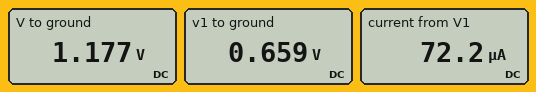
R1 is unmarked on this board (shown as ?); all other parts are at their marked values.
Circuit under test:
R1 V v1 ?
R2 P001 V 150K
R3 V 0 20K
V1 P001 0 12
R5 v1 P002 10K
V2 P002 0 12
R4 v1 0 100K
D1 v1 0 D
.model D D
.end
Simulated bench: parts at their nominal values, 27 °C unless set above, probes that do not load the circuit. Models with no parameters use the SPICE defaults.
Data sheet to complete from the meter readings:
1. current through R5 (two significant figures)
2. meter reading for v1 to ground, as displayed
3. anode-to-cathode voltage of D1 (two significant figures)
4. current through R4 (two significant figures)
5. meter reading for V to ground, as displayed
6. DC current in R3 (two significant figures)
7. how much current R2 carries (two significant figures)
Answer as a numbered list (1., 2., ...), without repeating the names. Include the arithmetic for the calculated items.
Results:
1. (12 V - 659 mV) / 10 kΩ = 1.1 mA
2. 0.659 V
3. 659 mV = 660 mV
4. (659 mV) / 100 kΩ = 6.6 µA
5. 1.177 V
6. (1.177 V) / 20 kΩ = 59 µA
7. (12 V - 1.177 V) / 150 kΩ = 72 µA
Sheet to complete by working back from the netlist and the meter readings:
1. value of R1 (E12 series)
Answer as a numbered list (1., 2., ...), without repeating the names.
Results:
1. 39 kΩ
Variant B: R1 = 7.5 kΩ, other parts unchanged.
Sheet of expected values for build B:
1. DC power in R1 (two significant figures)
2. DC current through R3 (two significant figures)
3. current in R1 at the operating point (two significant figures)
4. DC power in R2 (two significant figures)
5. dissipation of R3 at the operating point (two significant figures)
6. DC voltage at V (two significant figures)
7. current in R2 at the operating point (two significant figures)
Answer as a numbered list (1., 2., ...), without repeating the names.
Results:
1. 6.7 µW
2. 44 µA
3. 30 µA
4. 820 µW
5. 39 µW
6. 880 mV
7. 74 µA
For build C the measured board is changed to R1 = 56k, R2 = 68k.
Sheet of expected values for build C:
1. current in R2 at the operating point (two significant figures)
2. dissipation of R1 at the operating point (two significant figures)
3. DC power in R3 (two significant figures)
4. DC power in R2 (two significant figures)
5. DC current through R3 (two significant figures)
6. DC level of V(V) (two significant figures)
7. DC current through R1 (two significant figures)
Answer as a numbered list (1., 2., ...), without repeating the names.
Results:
1. 140 µA
2. 47 µW
3. 260 µW
4. 1.4 mW
5. 110 µA
6. 2.3 V
7. 29 µA
